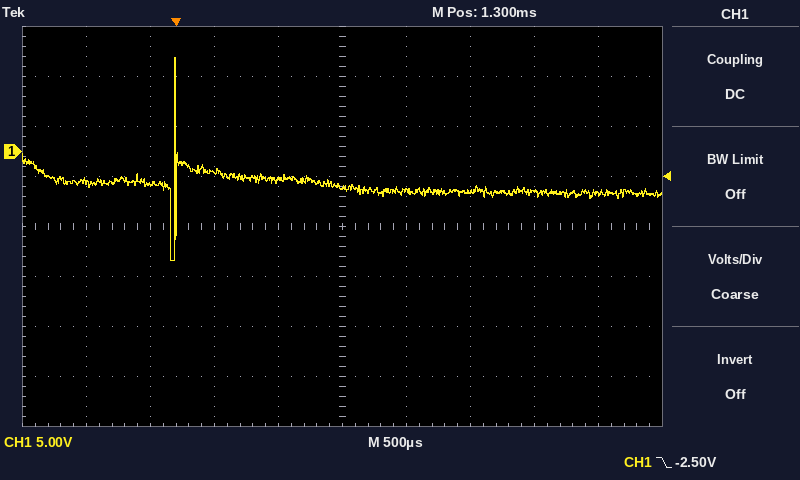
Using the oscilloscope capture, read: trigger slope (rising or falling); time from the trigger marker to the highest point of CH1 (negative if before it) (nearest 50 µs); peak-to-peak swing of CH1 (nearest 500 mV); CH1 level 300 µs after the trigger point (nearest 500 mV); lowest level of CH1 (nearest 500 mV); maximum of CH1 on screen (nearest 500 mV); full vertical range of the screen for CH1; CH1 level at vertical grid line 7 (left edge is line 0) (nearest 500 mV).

falling
0 µs
20.5 V
-2.0 V
-11.0 V
9.5 V
40 V
-4.0 V
